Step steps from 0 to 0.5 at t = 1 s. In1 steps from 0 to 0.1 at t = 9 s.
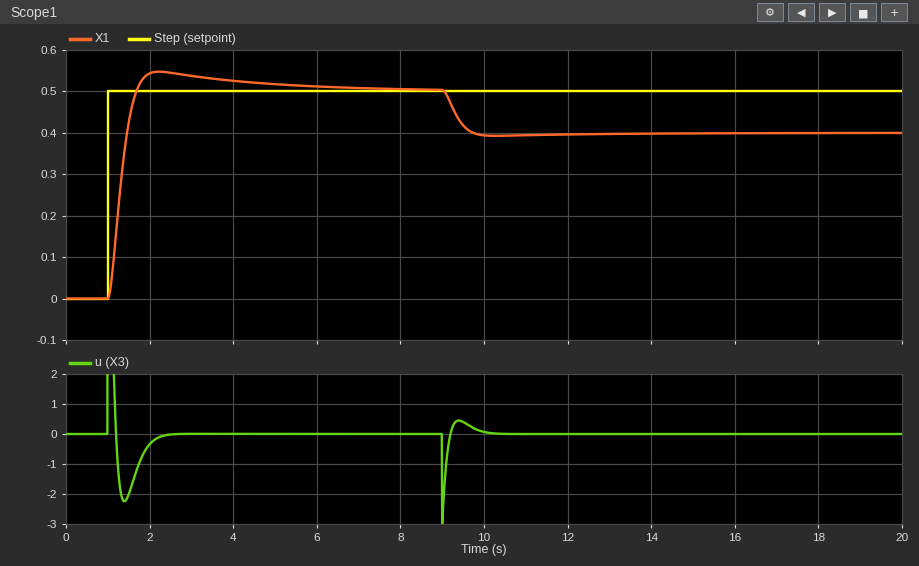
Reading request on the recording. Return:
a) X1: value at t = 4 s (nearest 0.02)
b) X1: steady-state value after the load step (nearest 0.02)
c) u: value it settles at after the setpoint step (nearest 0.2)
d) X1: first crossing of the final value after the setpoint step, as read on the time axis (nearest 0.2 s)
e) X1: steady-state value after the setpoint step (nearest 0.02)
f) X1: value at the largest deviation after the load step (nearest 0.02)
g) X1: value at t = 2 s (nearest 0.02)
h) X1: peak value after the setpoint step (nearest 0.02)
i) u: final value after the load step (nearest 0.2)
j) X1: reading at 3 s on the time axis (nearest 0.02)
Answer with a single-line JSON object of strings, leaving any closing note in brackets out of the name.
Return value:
{"X1: value at t = 4 s": "0.52", "X1: steady-state value after the load step": "0.40", "u: value it settles at after the setpoint step": "0.0", "X1: first crossing of the final value after the setpoint step, as read on the time axis": "1.6 s", "X1: steady-state value after the setpoint step": "0.50", "X1: value at the largest deviation after the load step": "0.40", "X1: value at t = 2 s": "0.54", "X1: peak value after the setpoint step": "0.54", "u: final value after the load step": "0.0", "X1: reading at 3 s on the time axis": "0.54"}
